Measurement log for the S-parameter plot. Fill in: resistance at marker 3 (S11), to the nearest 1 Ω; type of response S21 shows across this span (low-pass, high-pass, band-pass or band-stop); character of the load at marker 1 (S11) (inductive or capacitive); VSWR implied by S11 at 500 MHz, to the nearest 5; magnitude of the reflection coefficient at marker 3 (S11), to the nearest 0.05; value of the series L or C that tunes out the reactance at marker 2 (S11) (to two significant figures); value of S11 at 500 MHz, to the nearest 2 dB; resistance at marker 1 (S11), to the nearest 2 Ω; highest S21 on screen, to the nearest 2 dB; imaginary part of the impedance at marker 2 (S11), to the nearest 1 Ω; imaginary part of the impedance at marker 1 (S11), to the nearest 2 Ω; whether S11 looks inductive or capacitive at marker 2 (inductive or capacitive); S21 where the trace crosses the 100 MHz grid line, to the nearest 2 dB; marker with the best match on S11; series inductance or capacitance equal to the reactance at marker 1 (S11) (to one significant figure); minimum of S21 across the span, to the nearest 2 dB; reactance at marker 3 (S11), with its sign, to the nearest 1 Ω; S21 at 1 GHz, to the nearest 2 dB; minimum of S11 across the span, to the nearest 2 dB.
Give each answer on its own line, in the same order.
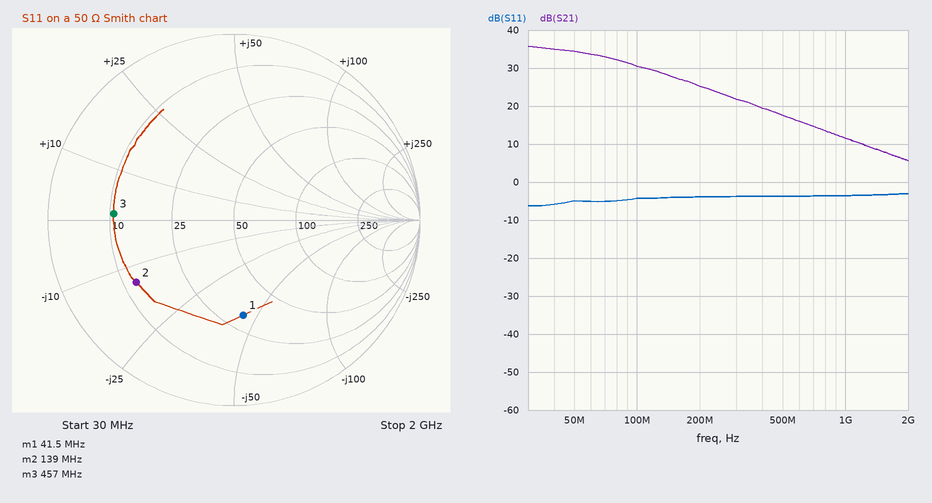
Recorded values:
11 Ω
low-pass
capacitive
5
0.65
16 nH
-4 dB
32 Ω
36 dB
-14 Ω
-44 Ω
capacitive
30 dB
marker 1
90 pF
6 dB
+1 Ω
12 dB
-6 dB
